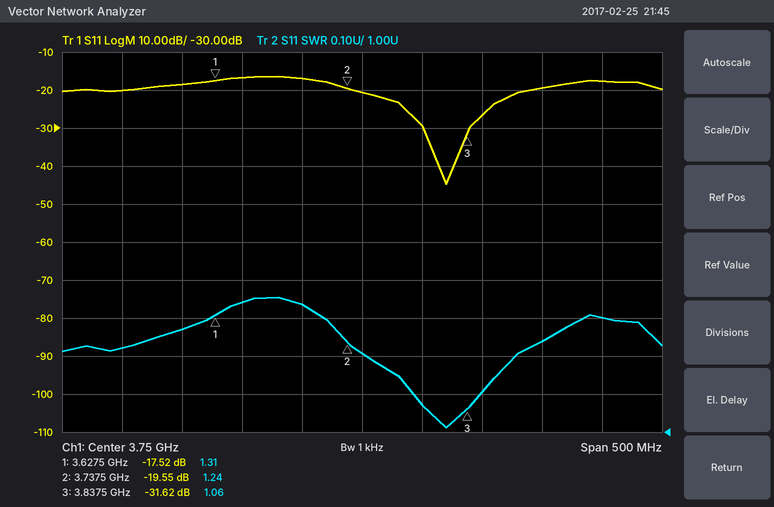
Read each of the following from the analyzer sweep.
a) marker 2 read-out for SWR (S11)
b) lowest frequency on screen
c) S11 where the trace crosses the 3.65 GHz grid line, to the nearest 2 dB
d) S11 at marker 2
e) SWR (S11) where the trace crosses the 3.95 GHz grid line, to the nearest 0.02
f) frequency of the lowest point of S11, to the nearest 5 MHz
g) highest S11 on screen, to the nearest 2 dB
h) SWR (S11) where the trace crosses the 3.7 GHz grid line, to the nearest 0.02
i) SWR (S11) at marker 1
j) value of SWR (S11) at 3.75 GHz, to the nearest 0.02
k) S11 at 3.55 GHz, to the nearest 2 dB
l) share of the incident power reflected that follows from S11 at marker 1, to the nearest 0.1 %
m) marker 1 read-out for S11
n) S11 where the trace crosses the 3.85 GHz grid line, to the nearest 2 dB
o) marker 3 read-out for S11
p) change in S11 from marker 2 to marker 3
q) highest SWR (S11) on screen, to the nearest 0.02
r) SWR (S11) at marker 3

1.24
3.5 GHz
-16 dB
-19.55 dB
1.30
3.820 GHz
-16 dB
1.34
1.31
1.20
-20 dB
1.8 %
-17.52 dB
-26 dB
-31.62 dB
-12.07 dB
1.36
1.06
